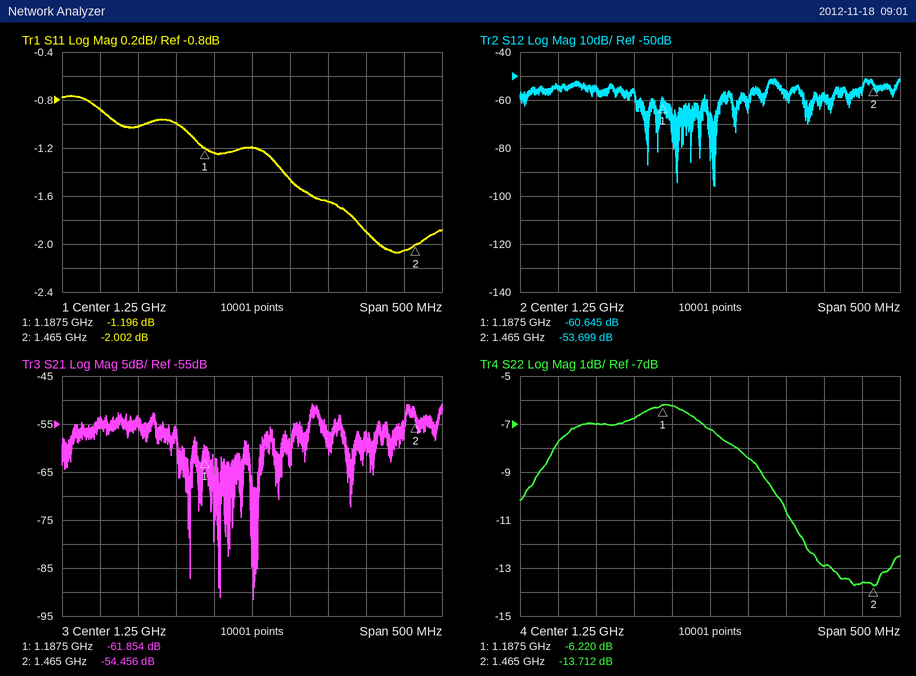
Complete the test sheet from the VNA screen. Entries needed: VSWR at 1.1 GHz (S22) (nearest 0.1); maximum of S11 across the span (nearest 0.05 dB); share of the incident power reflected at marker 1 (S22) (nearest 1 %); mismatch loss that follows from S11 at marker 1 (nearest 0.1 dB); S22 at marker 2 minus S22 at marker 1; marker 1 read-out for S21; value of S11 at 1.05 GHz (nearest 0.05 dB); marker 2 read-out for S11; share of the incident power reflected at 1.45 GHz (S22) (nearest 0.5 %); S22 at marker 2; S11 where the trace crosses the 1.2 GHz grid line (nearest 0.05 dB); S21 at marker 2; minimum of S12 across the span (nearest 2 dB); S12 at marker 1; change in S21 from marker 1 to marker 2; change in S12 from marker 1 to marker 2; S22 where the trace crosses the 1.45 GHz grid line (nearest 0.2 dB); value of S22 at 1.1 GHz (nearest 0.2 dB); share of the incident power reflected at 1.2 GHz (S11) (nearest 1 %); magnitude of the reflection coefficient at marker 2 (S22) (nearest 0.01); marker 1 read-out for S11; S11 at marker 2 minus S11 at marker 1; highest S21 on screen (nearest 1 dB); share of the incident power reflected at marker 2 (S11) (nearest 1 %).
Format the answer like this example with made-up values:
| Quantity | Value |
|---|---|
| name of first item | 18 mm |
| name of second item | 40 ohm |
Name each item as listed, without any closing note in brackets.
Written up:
| Quantity | Value |
|---|---|
| VSWR at 1.1 GHz (S22) | 2.6 |
| maximum of S11 across the span | -0.75 dB |
| share of the incident power reflected at marker 1 (S22) | 24 % |
| mismatch loss that follows from S11 at marker 1 | 6.2 dB |
| S22 at marker 2 minus S22 at marker 1 | -7.492 dB |
| marker 1 read-out for S21 | -61.854 dB |
| value of S11 at 1.05 GHz | -0.90 dB |
| marker 2 read-out for S11 | -2.002 dB |
| share of the incident power reflected at 1.45 GHz (S22) | 4.5 % |
| S22 at marker 2 | -13.712 dB |
| S11 where the trace crosses the 1.2 GHz grid line | -1.25 dB |
| S21 at marker 2 | -54.456 dB |
| minimum of S12 across the span | -96 dB |
| S12 at marker 1 | -60.645 dB |
| change in S21 from marker 1 to marker 2 | 7.398 dB |
| change in S12 from marker 1 to marker 2 | 6.946 dB |
| S22 where the trace crosses the 1.45 GHz grid line | -13.6 dB |
| value of S22 at 1.1 GHz | -7.0 dB |
| share of the incident power reflected at 1.2 GHz (S11) | 75 % |
| magnitude of the reflection coefficient at marker 2 (S22) | 0.21 |
| marker 1 read-out for S11 | -1.196 dB |
| S11 at marker 2 minus S11 at marker 1 | -0.806 dB |
| highest S21 on screen | -51 dB |
| share of the incident power reflected at marker 2 (S11) | 63 % |
